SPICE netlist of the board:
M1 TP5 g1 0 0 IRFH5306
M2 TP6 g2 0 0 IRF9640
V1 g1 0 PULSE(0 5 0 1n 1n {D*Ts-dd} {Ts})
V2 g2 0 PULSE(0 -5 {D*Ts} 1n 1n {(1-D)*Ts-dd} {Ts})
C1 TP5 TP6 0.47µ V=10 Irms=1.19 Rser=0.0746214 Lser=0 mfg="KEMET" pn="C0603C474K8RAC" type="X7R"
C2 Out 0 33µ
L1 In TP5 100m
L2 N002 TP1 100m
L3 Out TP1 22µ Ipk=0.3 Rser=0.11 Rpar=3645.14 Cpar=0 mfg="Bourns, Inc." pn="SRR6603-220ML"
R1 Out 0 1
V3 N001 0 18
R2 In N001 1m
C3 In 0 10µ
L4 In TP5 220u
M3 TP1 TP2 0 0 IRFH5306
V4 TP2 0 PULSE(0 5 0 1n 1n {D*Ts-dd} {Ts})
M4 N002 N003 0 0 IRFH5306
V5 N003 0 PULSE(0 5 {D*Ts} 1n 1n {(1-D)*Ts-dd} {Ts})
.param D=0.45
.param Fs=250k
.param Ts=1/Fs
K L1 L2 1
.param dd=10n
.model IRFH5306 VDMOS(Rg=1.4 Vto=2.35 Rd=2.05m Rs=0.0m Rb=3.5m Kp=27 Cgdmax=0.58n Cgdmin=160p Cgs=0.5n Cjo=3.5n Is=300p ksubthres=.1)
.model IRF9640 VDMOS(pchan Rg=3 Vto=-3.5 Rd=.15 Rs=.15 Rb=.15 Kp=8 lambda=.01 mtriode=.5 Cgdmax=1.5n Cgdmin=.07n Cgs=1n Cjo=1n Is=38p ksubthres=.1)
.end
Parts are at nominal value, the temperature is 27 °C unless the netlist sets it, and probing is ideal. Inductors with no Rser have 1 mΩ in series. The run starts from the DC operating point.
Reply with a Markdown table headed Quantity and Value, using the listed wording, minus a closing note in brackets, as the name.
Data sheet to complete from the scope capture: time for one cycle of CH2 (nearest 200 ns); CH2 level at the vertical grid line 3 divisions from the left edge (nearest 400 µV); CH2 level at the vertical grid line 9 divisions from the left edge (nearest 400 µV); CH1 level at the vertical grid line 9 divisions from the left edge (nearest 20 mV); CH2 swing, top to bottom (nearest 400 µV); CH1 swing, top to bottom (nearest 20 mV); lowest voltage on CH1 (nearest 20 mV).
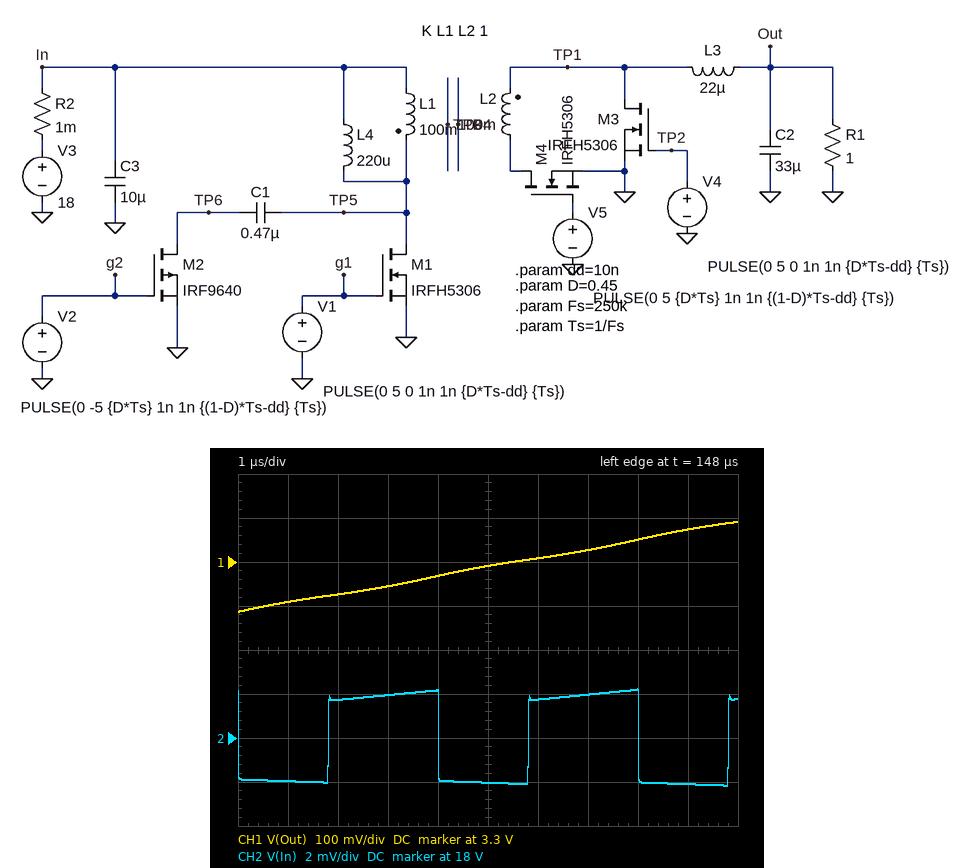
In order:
| Quantity | Value |
|---|---|
| time for one cycle of CH2 | 4.0 µs |
| CH2 level at the vertical grid line 3 divisions from the left edge | 18.0000 V |
| CH2 level at the vertical grid line 9 divisions from the left edge | 17.9960 V |
| CH1 level at the vertical grid line 9 divisions from the left edge | 3.38 V |
| CH2 swing, top to bottom | 4.4 mV |
| CH1 swing, top to bottom | 200 mV |
| lowest voltage on CH1 | 3.18 V |
